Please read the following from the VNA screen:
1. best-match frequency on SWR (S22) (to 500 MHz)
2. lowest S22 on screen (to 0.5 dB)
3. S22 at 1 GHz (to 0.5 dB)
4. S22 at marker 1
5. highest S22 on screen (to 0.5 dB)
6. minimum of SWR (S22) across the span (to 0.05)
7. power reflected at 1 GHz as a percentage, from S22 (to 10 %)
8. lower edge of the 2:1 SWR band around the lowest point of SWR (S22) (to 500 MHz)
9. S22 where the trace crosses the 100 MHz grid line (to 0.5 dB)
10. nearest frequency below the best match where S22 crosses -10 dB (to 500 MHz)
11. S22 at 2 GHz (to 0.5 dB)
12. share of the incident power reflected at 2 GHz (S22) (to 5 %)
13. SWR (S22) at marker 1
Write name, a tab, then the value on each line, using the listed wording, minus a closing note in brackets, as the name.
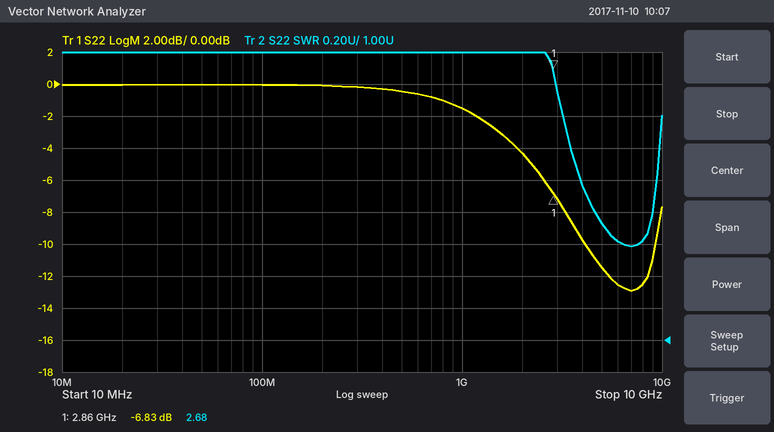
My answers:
best-match frequency on SWR (S22)	7.0 GHz
lowest S22 on screen	-13.0 dB
S22 at 1 GHz	-1.5 dB
S22 at marker 1	-6.83 dB
highest S22 on screen	0.0 dB
minimum of SWR (S22) across the span	1.60
power reflected at 1 GHz as a percentage, from S22	70 %
lower edge of the 2:1 SWR band around the lowest point of SWR (S22)	4.0 GHz
S22 where the trace crosses the 100 MHz grid line	0.0 dB
nearest frequency below the best match where S22 crosses -10 dB	4.0 GHz
S22 at 2 GHz	-4.5 dB
share of the incident power reflected at 2 GHz (S22)	35 %
SWR (S22) at marker 1	2.68
